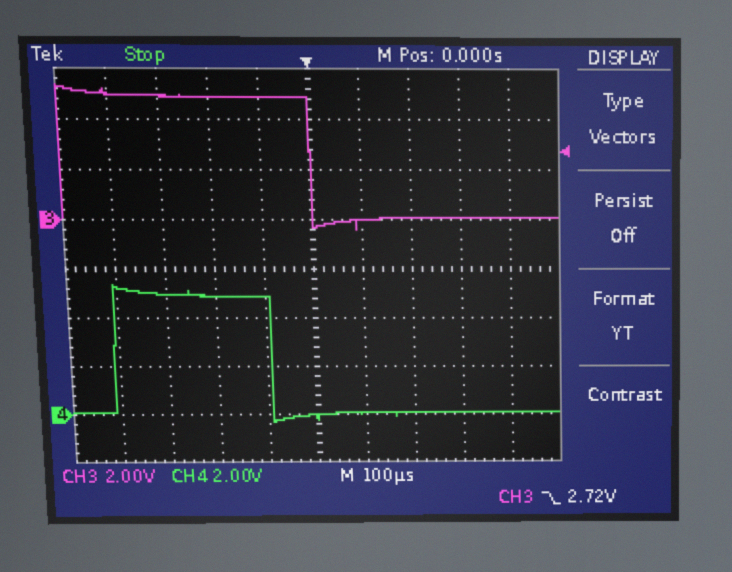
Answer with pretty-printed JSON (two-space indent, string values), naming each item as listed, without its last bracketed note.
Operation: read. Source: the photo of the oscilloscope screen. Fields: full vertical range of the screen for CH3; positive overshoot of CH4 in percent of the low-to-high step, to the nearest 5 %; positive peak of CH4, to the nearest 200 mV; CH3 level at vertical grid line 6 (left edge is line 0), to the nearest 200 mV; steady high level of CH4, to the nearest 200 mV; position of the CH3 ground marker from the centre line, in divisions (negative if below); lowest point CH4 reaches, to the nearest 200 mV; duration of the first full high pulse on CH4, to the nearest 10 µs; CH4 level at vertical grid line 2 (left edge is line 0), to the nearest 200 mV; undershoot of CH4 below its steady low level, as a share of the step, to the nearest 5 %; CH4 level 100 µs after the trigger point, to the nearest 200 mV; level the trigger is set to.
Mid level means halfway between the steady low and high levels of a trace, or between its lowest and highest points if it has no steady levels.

{
  "full vertical range of the screen for CH3": "16 V",
  "positive overshoot of CH4 in percent of the low-to-high step, to the nearest 5 %": "10 %",
  "positive peak of CH4, to the nearest 200 mV": "5.4 V",
  "CH3 level at vertical grid line 6 (left edge is line 0), to the nearest 200 mV": "0.0 V",
  "steady high level of CH4, to the nearest 200 mV": "5.0 V",
  "position of the CH3 ground marker from the centre line, in divisions": "+1.0 div",
  "lowest point CH4 reaches, to the nearest 200 mV": "-400 mV",
  "duration of the first full high pulse on CH4, to the nearest 10 µs": "320 µs",
  "CH4 level at vertical grid line 2 (left edge is line 0), to the nearest 200 mV": "5.0 V",
  "undershoot of CH4 below its steady low level, as a share of the step, to the nearest 5 %": "10 %",
  "CH4 level 100 µs after the trigger point, to the nearest 200 mV": "0.0 V",
  "level the trigger is set to": "2.72 V"
}
